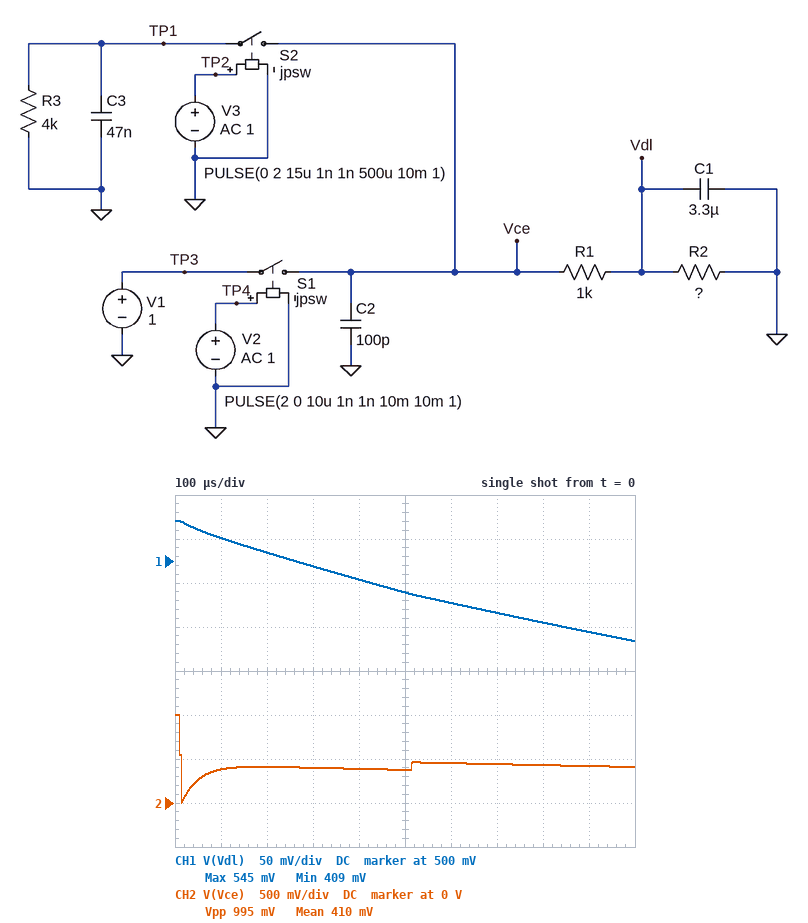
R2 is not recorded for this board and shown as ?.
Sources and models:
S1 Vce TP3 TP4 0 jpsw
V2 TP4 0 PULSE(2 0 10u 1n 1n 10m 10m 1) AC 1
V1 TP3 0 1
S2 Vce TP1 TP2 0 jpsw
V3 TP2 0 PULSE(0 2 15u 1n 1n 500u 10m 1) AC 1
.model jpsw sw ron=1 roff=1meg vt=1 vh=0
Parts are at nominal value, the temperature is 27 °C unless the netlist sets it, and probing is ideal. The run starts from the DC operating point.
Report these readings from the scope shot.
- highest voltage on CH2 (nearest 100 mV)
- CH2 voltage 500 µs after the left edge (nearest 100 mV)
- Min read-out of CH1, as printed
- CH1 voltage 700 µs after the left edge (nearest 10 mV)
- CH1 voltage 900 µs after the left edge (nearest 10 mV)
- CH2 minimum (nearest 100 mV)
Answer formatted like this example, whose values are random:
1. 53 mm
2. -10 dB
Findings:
1. 1.0 V
2. 400 mV
3. 409 mV
4. 440 mV
5. 420 mV
6. 0 V
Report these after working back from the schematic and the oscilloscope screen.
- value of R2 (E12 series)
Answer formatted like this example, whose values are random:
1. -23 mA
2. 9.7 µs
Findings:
1. 1.2 kΩ
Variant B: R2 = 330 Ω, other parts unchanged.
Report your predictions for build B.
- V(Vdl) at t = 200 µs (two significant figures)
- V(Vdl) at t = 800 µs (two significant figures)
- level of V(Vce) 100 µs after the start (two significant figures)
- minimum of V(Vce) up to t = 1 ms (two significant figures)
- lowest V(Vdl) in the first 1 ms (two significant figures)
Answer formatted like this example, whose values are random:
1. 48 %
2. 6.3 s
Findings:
1. 200 mV
2. 120 mV
3. 170 mV
4. 4.7 mV
5. 97 mV
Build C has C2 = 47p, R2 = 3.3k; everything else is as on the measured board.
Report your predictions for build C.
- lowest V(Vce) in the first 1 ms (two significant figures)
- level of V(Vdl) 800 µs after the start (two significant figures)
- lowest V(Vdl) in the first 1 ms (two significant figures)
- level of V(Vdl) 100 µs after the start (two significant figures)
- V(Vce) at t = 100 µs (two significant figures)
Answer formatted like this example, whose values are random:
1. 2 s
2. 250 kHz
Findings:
1. 5.5 mV
2. 690 mV
3. 670 mV
4. 750 mV
5. 540 mV
